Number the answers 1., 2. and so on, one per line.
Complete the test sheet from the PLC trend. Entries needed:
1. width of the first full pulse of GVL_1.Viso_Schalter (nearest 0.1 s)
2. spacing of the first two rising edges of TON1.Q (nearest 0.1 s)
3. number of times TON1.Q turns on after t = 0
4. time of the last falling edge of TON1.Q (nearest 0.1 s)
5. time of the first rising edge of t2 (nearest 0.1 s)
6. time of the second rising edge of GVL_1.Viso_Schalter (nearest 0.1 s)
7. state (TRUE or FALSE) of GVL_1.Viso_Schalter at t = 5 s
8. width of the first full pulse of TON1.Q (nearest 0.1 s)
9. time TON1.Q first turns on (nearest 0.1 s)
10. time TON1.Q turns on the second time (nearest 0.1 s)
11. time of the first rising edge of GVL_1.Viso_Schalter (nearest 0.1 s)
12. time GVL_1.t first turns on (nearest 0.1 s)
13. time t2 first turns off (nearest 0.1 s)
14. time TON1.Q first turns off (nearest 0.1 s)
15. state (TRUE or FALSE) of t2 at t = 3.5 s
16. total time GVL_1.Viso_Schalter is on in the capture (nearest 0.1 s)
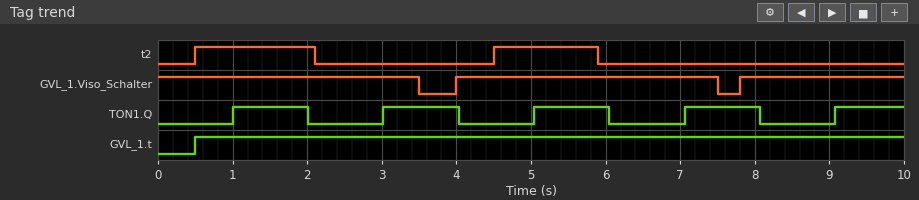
1. 3.5 s
2. 2.0 s
3. 5
4. 8.1 s
5. 0.5 s
6. 7.8 s
7. TRUE
8. 1.0 s
9. 1.0 s
10. 3.0 s
11. 4.0 s
12. 0.5 s
13. 2.1 s
14. 2.0 s
15. FALSE
16. 9.2 s
